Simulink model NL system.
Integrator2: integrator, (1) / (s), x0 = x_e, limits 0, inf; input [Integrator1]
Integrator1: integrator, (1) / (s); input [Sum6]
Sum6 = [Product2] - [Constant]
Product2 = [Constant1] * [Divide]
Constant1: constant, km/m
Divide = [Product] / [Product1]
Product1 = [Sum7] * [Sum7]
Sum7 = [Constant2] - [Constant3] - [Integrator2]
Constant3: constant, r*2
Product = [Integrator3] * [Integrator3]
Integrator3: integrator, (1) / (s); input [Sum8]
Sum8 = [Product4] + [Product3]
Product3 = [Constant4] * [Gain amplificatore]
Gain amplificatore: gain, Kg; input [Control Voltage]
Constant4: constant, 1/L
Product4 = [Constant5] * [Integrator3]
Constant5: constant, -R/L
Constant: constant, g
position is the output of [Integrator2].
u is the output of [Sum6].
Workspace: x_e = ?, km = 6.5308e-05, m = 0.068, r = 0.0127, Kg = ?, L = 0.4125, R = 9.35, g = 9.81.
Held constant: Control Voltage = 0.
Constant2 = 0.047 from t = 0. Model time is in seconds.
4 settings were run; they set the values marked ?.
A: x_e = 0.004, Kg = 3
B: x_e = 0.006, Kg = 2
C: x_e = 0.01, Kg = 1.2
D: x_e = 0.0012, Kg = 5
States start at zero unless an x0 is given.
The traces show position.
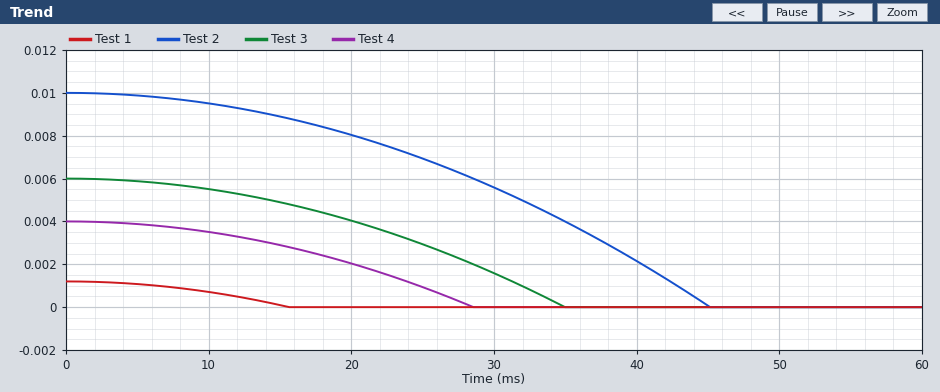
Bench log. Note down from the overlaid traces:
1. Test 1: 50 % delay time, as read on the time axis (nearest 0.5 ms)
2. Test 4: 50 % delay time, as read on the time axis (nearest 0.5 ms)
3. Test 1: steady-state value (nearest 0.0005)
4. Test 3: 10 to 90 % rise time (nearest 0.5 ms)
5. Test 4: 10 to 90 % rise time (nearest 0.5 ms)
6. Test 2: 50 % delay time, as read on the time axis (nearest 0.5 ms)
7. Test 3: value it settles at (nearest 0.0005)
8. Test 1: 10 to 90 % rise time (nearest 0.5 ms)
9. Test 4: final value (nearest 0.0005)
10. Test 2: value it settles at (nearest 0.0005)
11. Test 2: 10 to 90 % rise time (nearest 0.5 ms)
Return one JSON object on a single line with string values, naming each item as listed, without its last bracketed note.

{"Test 1: 50 % delay time, as read on the time axis": "11.0 ms", "Test 4: 50 % delay time, as read on the time axis": "20.0 ms", "Test 1: steady-state value": "0.0000", "Test 3: 10 to 90 % rise time": "22.0 ms", "Test 4: 10 to 90 % rise time": "18.0 ms", "Test 2: 50 % delay time, as read on the time axis": "32.0 ms", "Test 3: value it settles at": "0.0000", "Test 1: 10 to 90 % rise time": "10.0 ms", "Test 4: final value": "0.0000", "Test 2: value it settles at": "0.0000", "Test 2: 10 to 90 % rise time": "28.5 ms"}
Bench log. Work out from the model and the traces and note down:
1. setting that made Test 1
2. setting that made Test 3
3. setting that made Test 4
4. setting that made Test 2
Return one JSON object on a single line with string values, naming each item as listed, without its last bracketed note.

{"setting that made Test 1": "D", "setting that made Test 3": "B", "setting that made Test 4": "A", "setting that made Test 2": "C"}
